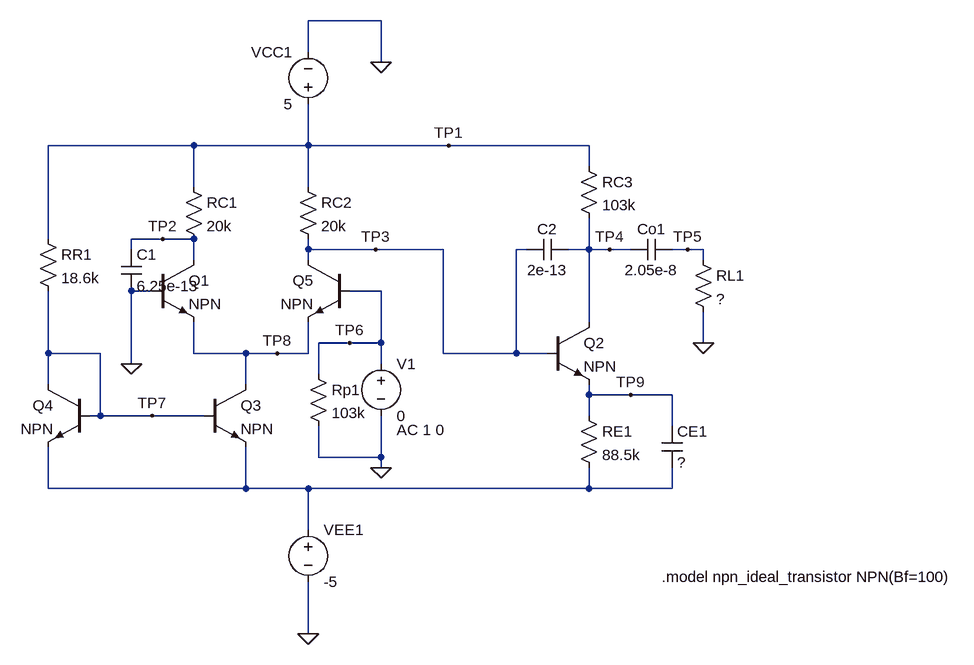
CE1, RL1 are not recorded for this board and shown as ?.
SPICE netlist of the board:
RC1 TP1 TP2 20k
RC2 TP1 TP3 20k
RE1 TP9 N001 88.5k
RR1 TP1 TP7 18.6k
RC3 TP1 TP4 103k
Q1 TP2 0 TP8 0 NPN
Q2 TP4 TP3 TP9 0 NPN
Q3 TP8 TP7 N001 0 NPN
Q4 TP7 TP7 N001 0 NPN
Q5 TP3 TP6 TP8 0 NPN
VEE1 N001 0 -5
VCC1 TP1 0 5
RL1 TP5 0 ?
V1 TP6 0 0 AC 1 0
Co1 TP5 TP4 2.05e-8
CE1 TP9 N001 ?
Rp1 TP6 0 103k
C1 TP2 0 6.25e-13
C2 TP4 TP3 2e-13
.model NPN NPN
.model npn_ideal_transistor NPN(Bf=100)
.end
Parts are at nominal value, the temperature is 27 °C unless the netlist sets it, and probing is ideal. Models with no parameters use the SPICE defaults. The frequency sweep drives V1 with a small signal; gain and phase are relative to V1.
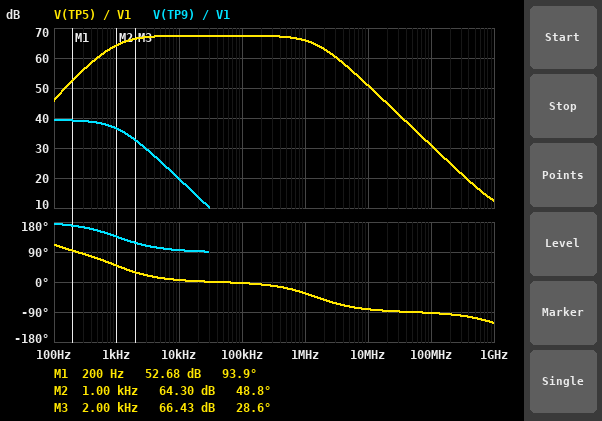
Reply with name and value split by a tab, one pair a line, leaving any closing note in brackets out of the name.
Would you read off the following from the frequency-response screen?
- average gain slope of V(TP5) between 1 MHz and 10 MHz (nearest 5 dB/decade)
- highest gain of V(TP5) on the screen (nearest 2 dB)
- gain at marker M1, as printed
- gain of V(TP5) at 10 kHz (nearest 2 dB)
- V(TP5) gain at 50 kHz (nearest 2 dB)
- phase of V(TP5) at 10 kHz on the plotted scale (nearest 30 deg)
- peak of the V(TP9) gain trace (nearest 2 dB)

average gain slope of V(TP5) between 1 MHz and 10 MHz	-15 dB/decade
highest gain of V(TP5) on the screen	68 dB
gain at marker M1, as printed	52.68 dB
gain of V(TP5) at 10 kHz	68 dB
V(TP5) gain at 50 kHz	68 dB
phase of V(TP5) at 10 kHz on the plotted scale	0 deg
peak of the V(TP9) gain trace	40 dB
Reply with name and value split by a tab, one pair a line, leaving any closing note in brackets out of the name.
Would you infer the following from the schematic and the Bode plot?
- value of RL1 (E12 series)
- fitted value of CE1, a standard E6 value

value of RL1	22 kΩ
fitted value of CE1, a standard E6 value	220 nF
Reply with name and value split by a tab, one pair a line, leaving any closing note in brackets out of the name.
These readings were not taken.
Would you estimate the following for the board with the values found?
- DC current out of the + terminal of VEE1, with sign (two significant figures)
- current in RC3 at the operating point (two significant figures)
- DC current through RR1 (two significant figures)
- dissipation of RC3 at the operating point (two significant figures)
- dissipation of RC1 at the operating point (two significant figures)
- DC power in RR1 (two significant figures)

DC current out of the + terminal of VEE1, with sign	-1.0 mA
current in RC3 at the operating point	50 µA
DC current through RR1	500 µA
dissipation of RC3 at the operating point	260 µW
dissipation of RC1 at the operating point	1.2 mW
DC power in RR1	4.6 mW
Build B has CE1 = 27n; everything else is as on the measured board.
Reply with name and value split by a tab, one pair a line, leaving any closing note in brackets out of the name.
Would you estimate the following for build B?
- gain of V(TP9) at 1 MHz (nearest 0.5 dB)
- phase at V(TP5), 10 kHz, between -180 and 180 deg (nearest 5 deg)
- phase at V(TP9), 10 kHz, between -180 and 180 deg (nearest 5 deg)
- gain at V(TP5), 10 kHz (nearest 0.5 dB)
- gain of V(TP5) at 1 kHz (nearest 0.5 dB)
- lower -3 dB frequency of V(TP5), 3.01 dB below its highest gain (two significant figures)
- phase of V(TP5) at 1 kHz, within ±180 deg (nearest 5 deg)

gain of V(TP9) at 1 MHz	-4.0 dB
phase at V(TP5), 10 kHz, between -180 and 180 deg	40 deg
phase at V(TP9), 10 kHz, between -180 and 180 deg	130 deg
gain at V(TP5), 10 kHz	65.0 dB
gain of V(TP5) at 1 kHz	49.0 dB
lower -3 dB frequency of V(TP5), 3.01 dB below its highest gain	8.3 kHz
phase of V(TP5) at 1 kHz, within ±180 deg	85 deg
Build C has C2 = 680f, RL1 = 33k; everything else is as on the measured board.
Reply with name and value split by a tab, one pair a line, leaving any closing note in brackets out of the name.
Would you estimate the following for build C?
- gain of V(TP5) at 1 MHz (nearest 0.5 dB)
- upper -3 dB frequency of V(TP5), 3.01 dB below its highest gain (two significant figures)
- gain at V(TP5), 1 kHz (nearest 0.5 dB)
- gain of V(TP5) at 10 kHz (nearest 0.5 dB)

gain of V(TP5) at 1 MHz	60.0 dB
upper -3 dB frequency of V(TP5), 3.01 dB below its highest gain	320 kHz
gain at V(TP5), 1 kHz	67.0 dB
gain of V(TP5) at 10 kHz	70.0 dB
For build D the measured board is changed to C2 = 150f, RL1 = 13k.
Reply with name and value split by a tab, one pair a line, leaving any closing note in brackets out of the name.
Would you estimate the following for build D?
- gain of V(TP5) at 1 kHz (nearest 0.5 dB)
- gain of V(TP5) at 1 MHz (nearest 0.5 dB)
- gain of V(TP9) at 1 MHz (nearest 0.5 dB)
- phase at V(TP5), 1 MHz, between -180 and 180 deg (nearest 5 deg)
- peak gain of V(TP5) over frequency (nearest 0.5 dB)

gain of V(TP5) at 1 kHz	60.5 dB
gain of V(TP5) at 1 MHz	63.0 dB
gain of V(TP9) at 1 MHz	-21.0 dB
phase at V(TP5), 1 MHz, between -180 and 180 deg	-20 deg
peak gain of V(TP5) over frequency	63.5 dB
